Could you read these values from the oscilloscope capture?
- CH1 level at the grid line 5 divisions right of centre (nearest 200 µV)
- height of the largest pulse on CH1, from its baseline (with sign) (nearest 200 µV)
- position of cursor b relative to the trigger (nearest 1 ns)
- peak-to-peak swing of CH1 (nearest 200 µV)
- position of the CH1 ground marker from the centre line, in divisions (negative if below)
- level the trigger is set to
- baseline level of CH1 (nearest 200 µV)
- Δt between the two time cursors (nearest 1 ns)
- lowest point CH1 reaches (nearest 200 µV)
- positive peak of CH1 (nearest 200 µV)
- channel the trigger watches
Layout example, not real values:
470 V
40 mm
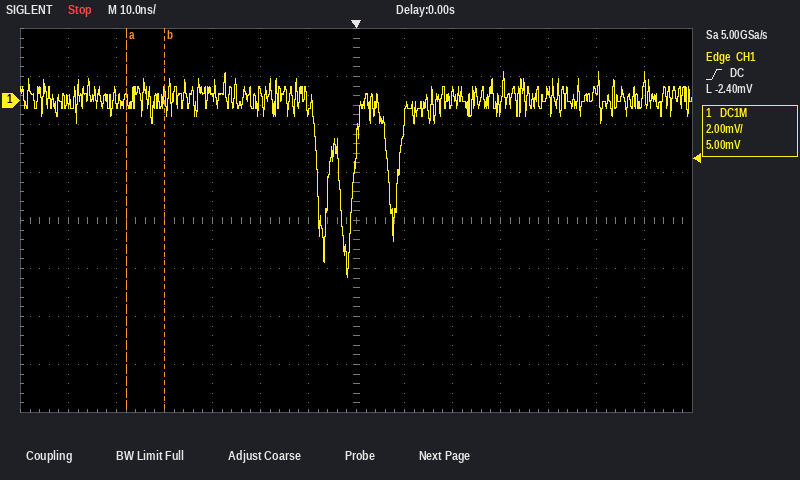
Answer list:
400 µV
-7.4 mV
-40 ns
8.6 mV
+2.5 div
-2.40 mV
0.0 mV
8 ns
-7.4 mV
1.2 mV
CH1
